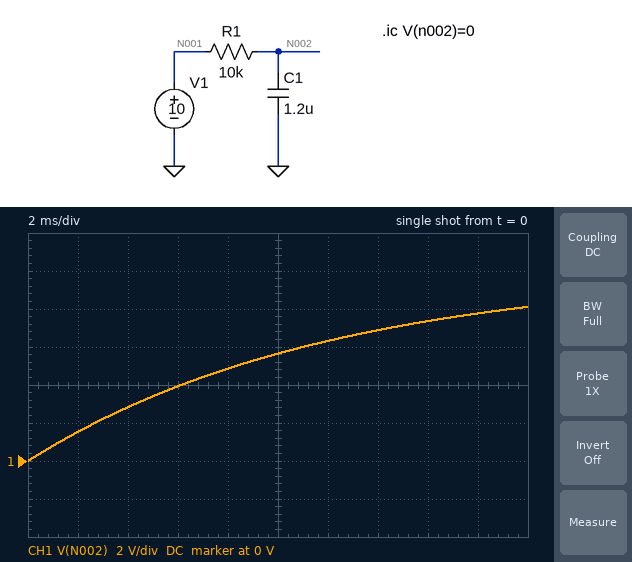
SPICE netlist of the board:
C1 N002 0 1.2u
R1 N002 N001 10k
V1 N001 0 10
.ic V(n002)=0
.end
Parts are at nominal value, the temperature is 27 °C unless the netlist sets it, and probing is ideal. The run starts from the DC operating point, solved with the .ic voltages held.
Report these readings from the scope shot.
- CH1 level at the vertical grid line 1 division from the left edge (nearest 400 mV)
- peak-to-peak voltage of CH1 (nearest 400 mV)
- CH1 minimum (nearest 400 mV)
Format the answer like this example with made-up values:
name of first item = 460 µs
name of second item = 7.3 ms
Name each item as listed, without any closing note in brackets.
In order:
CH1 level at the vertical grid line 1 division from the left edge = 1.6 V
peak-to-peak voltage of CH1 = 8.0 V
CH1 minimum = 0 V
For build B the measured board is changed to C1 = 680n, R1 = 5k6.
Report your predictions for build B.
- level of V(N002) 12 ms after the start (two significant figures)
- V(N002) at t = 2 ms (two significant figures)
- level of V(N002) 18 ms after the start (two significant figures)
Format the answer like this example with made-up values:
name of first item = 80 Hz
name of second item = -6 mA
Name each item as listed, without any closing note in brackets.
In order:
level of V(N002) 12 ms after the start = 9.6 V
V(N002) at t = 2 ms = 4.1 V
level of V(N002) 18 ms after the start = 9.9 V
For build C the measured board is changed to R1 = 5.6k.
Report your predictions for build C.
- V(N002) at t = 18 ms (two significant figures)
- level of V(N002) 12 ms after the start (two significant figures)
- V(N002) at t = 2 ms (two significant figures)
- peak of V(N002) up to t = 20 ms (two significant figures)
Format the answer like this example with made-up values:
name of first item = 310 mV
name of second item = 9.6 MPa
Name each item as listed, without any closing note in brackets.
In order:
V(N002) at t = 18 ms = 9.3 V
level of V(N002) 12 ms after the start = 8.3 V
V(N002) at t = 2 ms = 2.6 V
peak of V(N002) up to t = 20 ms = 9.5 V
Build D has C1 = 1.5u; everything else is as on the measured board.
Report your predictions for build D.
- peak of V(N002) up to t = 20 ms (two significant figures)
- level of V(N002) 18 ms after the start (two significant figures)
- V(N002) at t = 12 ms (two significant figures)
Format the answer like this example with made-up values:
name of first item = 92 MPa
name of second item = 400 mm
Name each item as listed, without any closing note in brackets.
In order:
peak of V(N002) up to t = 20 ms = 7.4 V
level of V(N002) 18 ms after the start = 7.0 V
V(N002) at t = 12 ms = 5.5 V
